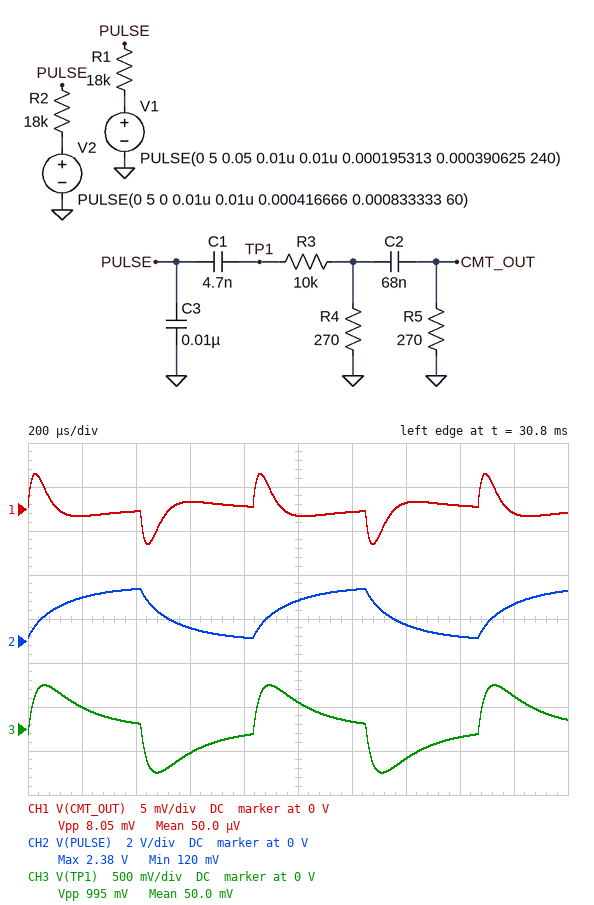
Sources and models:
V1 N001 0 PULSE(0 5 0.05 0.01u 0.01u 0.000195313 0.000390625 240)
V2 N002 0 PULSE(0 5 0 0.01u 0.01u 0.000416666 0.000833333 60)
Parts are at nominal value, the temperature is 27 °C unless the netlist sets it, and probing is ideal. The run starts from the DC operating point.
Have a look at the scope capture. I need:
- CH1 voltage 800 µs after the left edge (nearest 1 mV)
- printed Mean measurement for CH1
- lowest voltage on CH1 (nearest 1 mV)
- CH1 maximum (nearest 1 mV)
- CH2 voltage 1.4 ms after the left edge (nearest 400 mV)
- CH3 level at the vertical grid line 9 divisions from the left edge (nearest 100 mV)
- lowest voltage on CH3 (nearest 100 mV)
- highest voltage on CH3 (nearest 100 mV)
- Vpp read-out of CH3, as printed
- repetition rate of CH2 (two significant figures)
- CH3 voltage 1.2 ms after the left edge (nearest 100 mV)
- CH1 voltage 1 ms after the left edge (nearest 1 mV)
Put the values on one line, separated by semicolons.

0 V; 50.0 µV; -4 mV; 4 mV; 800 mV; 400 mV; -500 mV; 500 mV; 995 mV; 1.2 kHz; 100 mV; -1 mV
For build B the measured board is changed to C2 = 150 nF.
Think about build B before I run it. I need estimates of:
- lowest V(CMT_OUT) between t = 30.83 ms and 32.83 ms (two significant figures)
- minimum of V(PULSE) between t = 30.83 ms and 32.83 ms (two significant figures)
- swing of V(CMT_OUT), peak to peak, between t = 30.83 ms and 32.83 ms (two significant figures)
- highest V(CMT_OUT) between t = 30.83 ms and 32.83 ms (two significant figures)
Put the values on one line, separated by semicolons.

-5.5 mV; 130 mV; 11 mV; 5.5 mV
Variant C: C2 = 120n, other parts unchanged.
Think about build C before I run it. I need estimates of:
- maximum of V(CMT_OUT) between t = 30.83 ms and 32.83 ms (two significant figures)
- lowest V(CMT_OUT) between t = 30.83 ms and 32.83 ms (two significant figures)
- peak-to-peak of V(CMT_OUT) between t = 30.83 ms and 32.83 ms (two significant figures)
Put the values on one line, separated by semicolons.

5.1 mV; -5.1 mV; 10 mV
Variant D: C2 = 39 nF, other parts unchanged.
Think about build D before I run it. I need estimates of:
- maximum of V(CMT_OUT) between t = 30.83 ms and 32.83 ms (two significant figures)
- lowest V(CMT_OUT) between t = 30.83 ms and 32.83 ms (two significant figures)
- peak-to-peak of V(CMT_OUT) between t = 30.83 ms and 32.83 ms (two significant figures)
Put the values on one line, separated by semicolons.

3.1 mV; -3.1 mV; 6.1 mV
